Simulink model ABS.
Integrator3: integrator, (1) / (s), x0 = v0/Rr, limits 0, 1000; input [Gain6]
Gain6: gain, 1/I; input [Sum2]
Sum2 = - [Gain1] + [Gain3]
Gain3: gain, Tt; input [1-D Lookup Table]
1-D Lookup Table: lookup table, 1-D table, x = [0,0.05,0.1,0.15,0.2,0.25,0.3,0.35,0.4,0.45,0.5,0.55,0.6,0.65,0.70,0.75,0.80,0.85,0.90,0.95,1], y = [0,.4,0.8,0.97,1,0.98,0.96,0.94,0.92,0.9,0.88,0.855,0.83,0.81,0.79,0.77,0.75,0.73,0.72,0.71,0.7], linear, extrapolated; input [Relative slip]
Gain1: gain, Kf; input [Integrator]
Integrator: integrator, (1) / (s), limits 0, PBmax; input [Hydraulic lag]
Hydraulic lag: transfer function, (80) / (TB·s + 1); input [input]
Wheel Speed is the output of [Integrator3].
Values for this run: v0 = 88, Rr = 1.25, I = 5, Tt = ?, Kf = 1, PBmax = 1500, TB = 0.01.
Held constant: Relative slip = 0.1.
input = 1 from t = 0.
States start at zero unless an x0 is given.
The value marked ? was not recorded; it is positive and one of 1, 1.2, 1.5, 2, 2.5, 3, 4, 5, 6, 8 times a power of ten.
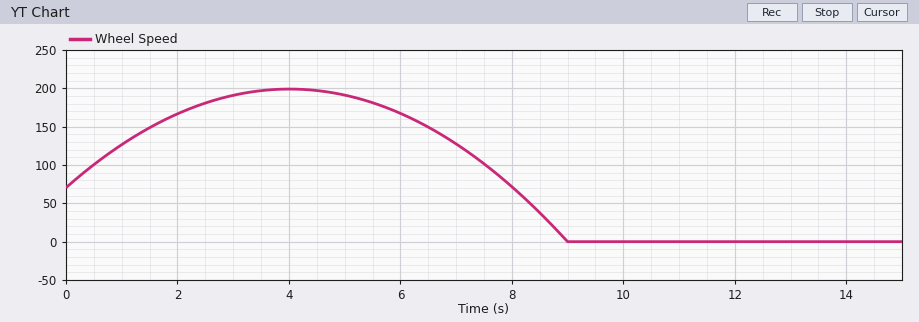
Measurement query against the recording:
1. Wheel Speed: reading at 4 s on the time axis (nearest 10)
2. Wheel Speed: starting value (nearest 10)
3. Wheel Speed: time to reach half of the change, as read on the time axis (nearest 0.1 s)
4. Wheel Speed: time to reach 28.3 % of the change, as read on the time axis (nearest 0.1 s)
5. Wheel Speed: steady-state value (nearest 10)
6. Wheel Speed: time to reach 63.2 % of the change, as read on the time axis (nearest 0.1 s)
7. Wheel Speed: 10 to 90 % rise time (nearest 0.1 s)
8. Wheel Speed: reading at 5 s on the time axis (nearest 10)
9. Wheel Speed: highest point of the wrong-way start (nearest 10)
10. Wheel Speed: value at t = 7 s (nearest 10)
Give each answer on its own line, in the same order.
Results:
200
70
8.5 s
8.3 s
0
8.7 s
0.8 s
190
200
130
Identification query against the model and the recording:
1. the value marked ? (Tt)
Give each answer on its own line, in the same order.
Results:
400
